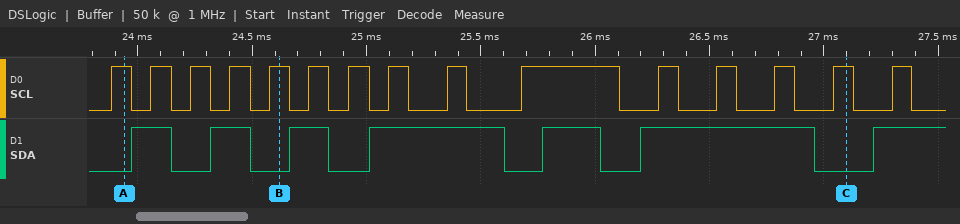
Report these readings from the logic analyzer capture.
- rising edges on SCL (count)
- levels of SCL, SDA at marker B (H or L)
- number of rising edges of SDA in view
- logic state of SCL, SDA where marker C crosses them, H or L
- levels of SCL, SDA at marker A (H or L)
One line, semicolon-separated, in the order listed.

15; SCL=H, SDA=L; 7; SCL=H, SDA=L; SCL=H, SDA=L
